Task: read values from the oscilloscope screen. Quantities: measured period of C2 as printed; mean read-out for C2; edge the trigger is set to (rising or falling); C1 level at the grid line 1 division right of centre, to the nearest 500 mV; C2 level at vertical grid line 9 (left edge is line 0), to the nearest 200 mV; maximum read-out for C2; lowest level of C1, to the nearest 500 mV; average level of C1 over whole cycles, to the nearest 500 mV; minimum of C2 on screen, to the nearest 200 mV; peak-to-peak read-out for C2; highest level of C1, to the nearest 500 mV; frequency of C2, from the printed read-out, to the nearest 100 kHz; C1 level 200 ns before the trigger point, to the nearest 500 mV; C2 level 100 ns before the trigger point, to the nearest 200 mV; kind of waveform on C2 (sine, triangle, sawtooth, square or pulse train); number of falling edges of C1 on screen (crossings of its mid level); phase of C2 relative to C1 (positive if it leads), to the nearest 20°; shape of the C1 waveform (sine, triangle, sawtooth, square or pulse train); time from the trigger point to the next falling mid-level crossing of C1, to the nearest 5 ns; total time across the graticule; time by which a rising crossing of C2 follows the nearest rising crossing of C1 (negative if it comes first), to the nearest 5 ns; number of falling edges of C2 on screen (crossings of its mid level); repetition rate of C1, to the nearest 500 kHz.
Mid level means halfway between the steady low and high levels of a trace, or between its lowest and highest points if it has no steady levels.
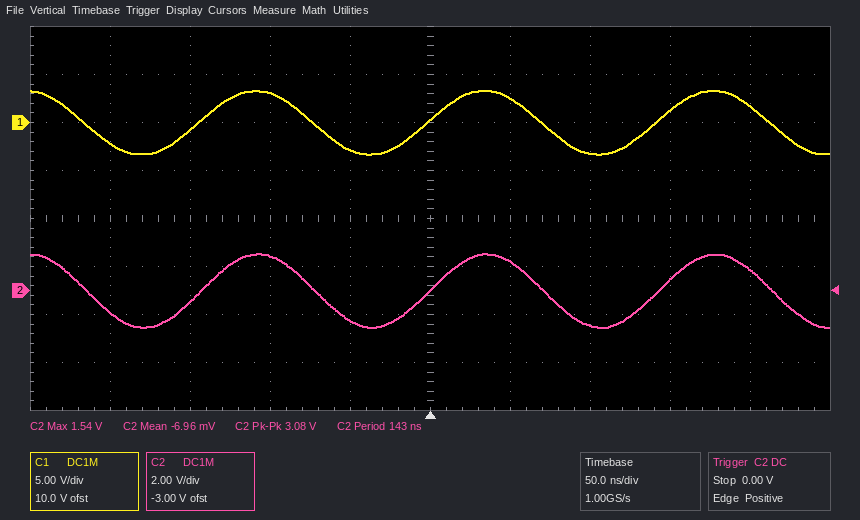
143 ns
-6.96 mV
rising
2.5 V
800 mV
1.54 V
-3.5 V
0.0 V
-1.6 V
3.08 V
3.5 V
7.0 MHz
-2.0 V
1.4 V
sine
4
0°
sine
70 ns
500 ns
0 ns
4
7.0 MHz
